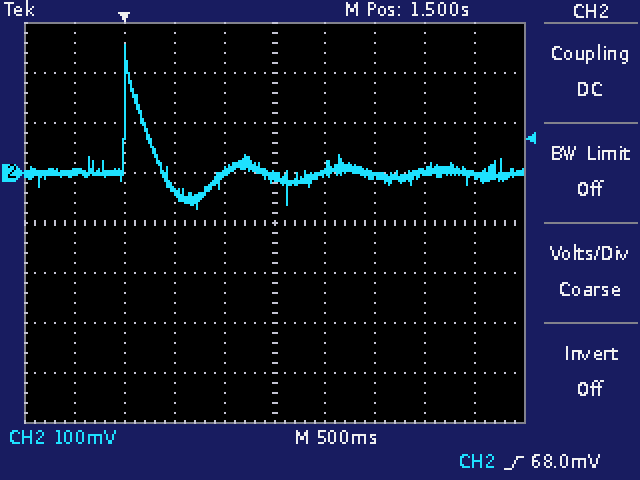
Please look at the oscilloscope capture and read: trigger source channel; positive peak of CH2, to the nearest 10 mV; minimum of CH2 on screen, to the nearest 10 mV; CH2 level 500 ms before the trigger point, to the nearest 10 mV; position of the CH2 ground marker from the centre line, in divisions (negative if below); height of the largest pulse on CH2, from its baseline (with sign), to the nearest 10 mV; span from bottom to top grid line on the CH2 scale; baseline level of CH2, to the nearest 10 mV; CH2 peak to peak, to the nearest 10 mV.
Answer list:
CH2
260 mV
-70 mV
0 mV
+1.0 div
+260 mV
800 mV
0 mV
330 mV
